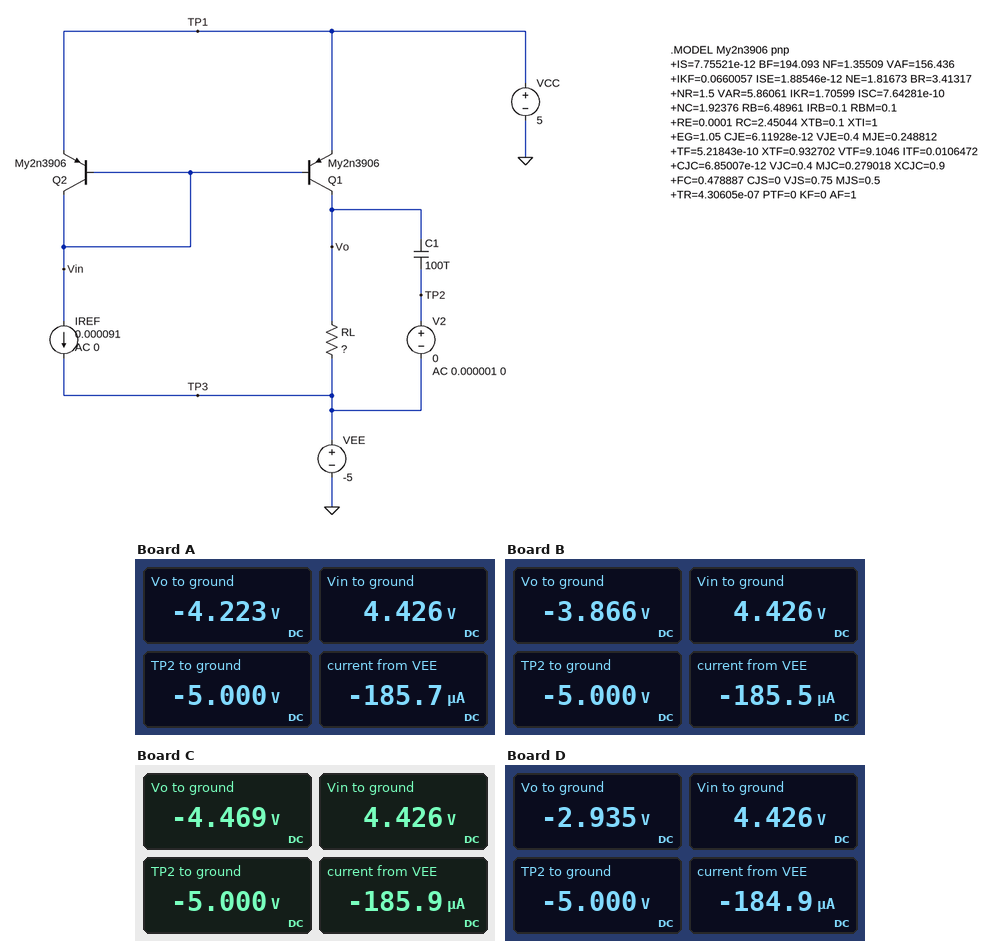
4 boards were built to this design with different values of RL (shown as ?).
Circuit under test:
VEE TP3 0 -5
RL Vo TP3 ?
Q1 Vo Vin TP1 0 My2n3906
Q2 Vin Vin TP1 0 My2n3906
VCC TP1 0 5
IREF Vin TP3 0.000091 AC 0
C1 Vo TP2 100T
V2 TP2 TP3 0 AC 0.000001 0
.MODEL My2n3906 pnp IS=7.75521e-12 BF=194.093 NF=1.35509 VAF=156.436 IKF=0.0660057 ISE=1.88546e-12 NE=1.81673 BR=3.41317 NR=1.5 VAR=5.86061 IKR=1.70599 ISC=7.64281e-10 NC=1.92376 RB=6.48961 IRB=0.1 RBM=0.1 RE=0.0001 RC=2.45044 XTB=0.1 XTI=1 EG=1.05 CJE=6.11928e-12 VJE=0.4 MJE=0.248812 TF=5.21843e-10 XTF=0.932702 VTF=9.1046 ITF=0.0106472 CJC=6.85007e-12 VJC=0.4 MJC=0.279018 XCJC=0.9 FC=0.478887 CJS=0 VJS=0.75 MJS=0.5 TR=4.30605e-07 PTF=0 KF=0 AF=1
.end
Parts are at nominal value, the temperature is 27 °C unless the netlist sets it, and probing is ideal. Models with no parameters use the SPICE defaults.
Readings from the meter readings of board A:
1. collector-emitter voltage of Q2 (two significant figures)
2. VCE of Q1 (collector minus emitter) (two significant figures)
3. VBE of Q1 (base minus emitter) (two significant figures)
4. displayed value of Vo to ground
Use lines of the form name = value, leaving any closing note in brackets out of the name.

collector-emitter voltage of Q2 = -570 mV
VCE of Q1 (collector minus emitter) = -9.2 V
VBE of Q1 (base minus emitter) = -570 mV
displayed value of Vo to ground = -4.223 V
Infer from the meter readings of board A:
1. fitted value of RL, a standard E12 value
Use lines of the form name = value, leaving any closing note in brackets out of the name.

fitted value of RL, a standard E12 value = 8.2 kΩ
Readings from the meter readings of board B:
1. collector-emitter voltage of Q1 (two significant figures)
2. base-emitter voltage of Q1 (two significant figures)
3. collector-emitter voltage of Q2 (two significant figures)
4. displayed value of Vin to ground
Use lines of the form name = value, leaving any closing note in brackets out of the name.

collector-emitter voltage of Q1 = -8.9 V
base-emitter voltage of Q1 = -570 mV
collector-emitter voltage of Q2 = -570 mV
displayed value of Vin to ground = 4.426 V
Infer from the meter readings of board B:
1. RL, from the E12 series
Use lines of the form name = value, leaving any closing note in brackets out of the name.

RL, from the E12 series = 12 kΩ
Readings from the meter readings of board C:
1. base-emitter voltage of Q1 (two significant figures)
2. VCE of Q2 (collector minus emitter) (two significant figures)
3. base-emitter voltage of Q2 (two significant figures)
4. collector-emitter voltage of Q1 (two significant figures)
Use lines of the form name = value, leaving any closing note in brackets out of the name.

base-emitter voltage of Q1 = -570 mV
VCE of Q2 (collector minus emitter) = -570 mV
base-emitter voltage of Q2 = -570 mV
collector-emitter voltage of Q1 = -9.5 V
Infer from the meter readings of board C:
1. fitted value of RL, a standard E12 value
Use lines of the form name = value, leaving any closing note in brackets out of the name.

fitted value of RL, a standard E12 value = 5.6 kΩ
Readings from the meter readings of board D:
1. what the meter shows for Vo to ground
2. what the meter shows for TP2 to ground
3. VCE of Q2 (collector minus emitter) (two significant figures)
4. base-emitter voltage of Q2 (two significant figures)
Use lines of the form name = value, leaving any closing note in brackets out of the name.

what the meter shows for Vo to ground = -2.935 V
what the meter shows for TP2 to ground = -5.000 V
VCE of Q2 (collector minus emitter) = -570 mV
base-emitter voltage of Q2 = -570 mV
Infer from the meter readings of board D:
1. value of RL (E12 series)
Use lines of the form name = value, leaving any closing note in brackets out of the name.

value of RL = 22 kΩ
